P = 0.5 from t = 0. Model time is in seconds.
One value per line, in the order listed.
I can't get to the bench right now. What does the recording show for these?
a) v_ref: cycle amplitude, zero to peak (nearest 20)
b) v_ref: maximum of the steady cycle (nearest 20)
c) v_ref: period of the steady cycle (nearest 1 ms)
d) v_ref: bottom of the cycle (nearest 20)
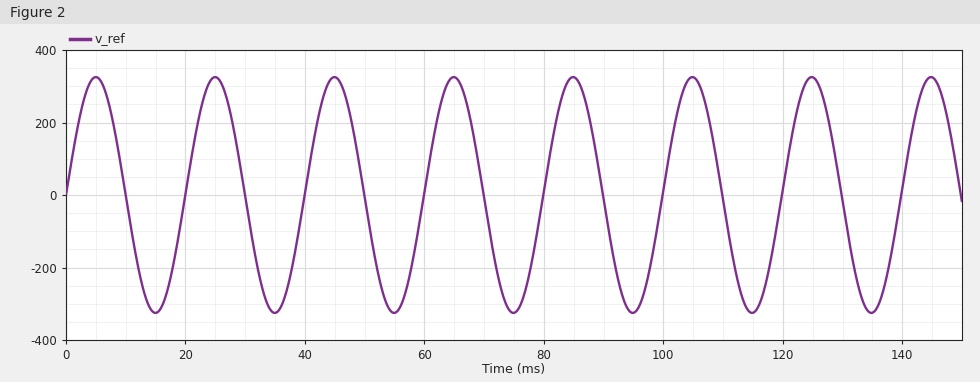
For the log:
320
320
20 ms
-320
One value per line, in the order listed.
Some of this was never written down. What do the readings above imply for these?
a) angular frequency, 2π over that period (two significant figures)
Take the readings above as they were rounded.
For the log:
0.31 rad/ms
